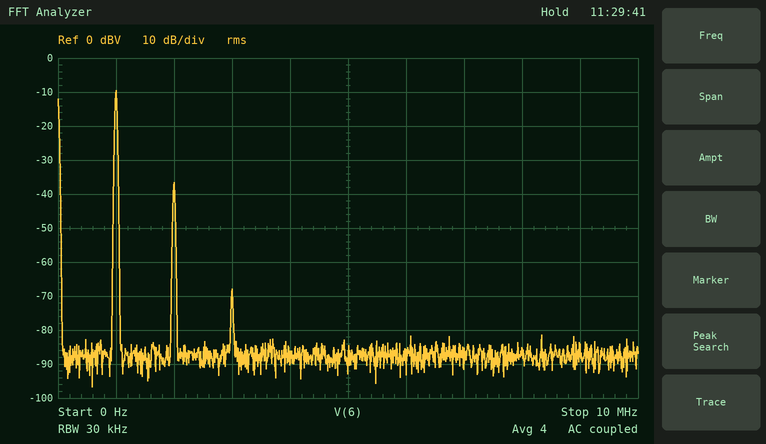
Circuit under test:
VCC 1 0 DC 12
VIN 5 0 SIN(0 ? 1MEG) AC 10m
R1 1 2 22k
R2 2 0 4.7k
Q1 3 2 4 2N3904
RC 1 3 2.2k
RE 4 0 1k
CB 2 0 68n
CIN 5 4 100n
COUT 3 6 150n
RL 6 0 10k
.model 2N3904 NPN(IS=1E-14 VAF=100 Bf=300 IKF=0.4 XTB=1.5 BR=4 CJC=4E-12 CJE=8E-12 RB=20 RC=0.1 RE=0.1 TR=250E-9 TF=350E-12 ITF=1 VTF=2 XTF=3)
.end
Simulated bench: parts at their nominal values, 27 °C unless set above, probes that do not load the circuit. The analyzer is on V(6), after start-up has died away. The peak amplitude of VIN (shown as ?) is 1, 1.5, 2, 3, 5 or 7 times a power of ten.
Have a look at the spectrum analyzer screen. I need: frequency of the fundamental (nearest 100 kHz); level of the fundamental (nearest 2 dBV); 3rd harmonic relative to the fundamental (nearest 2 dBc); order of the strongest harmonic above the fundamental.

1.0 MHz
-10 dBV
-58 dBc
2
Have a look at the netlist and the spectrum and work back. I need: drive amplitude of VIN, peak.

5 mV
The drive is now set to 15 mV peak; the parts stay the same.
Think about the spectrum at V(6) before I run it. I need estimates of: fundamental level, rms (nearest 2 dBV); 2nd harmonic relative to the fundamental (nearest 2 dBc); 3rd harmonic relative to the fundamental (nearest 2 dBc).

0 dBV
-18 dBc
-40 dBc
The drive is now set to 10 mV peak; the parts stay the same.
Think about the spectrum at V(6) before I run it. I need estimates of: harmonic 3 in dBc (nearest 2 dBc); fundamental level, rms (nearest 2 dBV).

-46 dBc
-4 dBV
